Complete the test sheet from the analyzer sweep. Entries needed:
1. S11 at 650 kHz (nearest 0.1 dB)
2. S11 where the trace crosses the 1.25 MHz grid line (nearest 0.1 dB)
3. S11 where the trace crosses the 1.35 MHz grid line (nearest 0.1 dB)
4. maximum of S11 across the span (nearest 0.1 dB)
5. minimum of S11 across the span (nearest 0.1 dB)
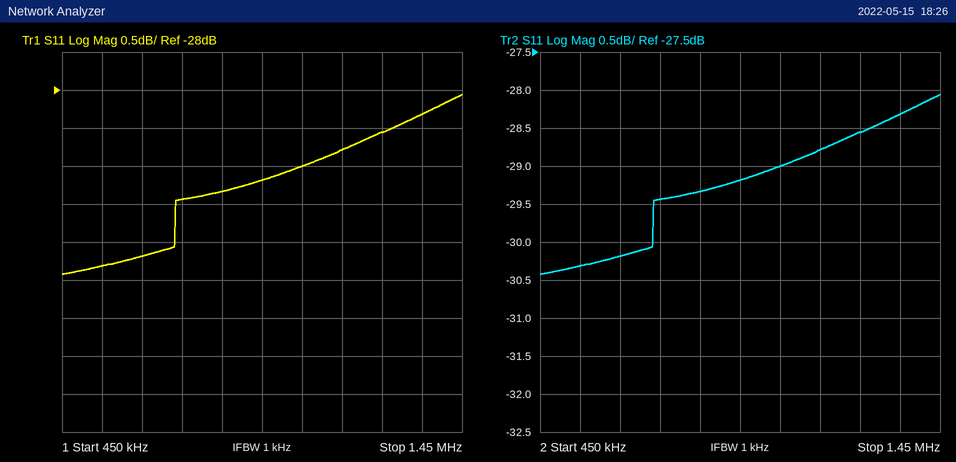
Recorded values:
-30.2 dB
-28.6 dB
-28.3 dB
-28.1 dB
-30.4 dB
